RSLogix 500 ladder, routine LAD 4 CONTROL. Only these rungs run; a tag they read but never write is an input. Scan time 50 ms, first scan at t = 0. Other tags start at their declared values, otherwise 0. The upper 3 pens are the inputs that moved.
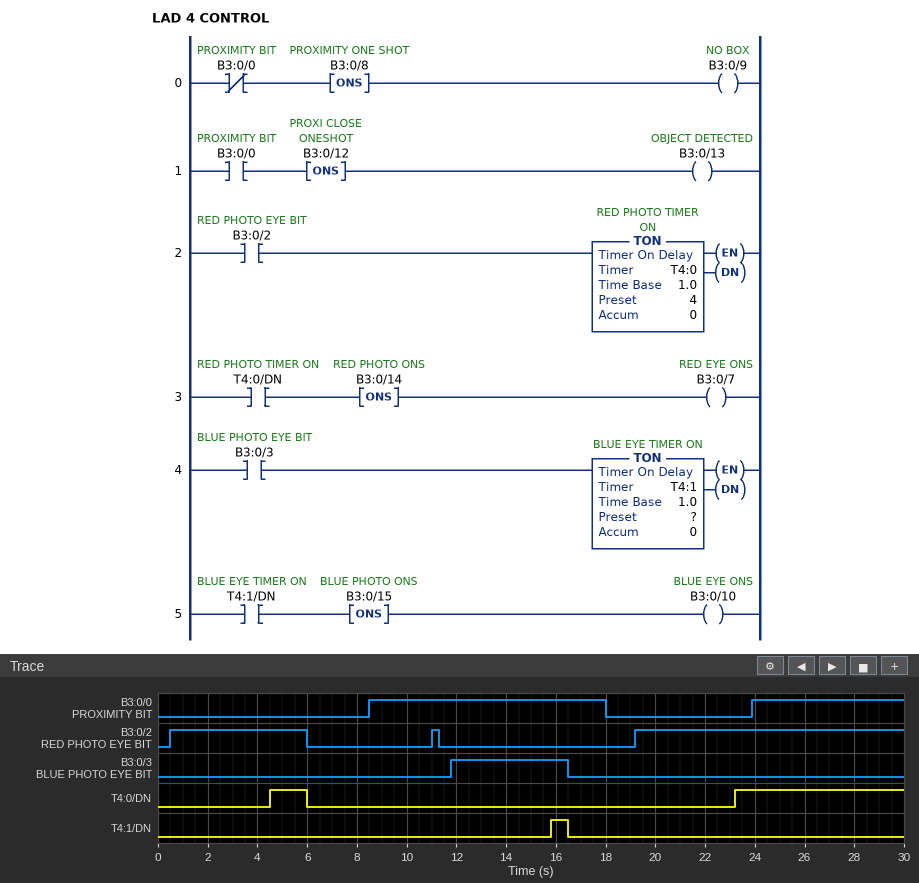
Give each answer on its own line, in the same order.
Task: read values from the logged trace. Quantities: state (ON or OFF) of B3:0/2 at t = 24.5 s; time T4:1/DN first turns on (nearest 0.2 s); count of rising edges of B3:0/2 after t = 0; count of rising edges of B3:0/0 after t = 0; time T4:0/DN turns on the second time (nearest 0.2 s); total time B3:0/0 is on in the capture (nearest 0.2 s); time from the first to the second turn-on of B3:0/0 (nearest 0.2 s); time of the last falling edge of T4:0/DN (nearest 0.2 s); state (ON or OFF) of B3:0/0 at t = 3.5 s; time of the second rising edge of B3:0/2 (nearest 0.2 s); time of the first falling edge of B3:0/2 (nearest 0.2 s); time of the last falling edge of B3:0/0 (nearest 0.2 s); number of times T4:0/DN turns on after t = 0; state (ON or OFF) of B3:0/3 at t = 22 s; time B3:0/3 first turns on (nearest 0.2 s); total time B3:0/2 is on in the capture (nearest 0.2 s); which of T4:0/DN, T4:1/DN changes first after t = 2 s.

ON
15.8 s
3
2
23.2 s
15.6 s
15.4 s
6.0 s
OFF
11.0 s
6.0 s
18.0 s
2
OFF
11.8 s
16.6 s
T4:0/DN
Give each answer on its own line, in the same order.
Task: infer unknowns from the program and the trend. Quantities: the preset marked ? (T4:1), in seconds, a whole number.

4 s
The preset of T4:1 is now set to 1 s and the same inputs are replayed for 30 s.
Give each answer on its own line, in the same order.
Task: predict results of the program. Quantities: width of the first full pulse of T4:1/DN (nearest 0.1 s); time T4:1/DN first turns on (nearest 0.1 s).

3.7 s
12.8 s
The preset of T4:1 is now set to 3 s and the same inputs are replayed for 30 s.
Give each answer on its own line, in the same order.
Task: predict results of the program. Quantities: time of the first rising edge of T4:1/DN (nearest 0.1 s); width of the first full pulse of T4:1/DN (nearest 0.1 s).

14.8 s
1.7 s
